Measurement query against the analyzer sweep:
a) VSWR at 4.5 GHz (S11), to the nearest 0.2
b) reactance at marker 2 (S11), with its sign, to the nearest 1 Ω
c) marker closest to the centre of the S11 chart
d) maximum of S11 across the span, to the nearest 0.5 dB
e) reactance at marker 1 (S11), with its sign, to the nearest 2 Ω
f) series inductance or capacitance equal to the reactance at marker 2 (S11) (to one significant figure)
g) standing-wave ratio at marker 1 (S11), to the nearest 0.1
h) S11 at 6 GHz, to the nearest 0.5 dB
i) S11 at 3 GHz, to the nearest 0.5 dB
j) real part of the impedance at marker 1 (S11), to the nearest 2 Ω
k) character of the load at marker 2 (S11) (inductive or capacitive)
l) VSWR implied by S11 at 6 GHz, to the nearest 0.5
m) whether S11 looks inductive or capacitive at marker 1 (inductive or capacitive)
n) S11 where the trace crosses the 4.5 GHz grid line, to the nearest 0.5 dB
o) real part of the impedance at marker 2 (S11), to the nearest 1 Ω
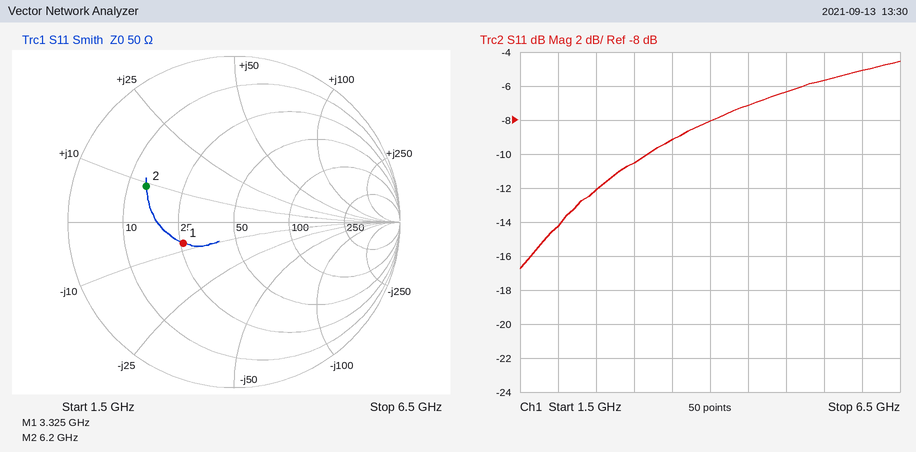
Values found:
2.6
+9 Ω
marker 1
-4.5 dB
-8 Ω
200 pH
2.0
-5.0 dB
-10.5 dB
26 Ω
inductive
3.5
capacitive
-7.0 dB
14 Ω
